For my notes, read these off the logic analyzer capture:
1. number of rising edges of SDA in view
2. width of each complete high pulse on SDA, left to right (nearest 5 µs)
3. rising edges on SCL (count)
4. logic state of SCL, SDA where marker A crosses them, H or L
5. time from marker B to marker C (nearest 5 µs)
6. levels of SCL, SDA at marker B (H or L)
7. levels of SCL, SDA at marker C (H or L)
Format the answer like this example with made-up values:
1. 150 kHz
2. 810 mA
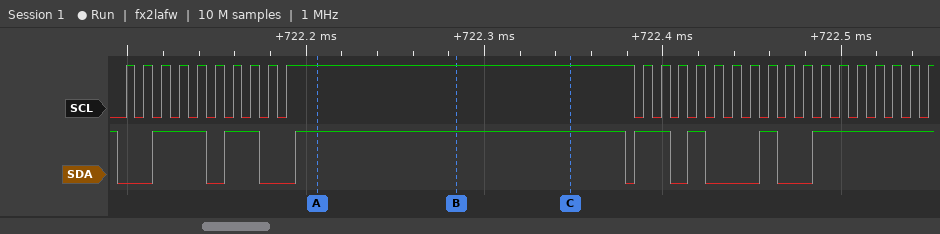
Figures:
1. 7
2. 30 µs, 20 µs, 185 µs, 20 µs, 10 µs, 10 µs
3. 27
4. SCL=H, SDA=H
5. 65 µs
6. SCL=H, SDA=H
7. SCL=H, SDA=H
